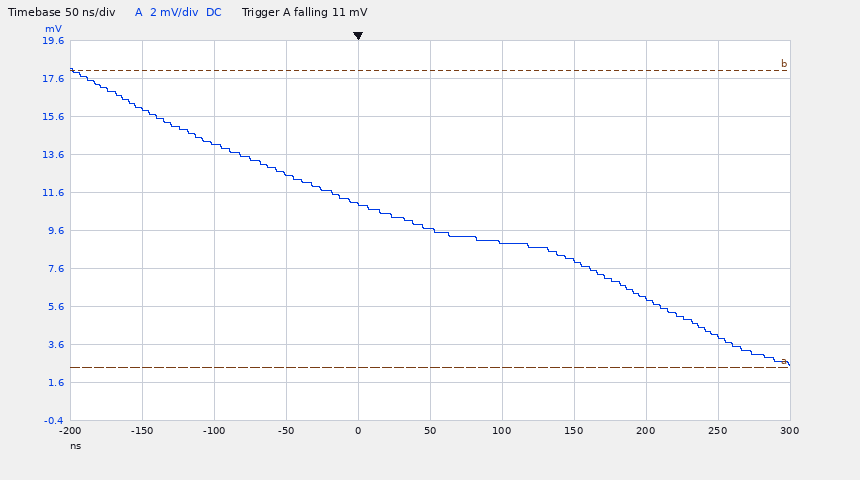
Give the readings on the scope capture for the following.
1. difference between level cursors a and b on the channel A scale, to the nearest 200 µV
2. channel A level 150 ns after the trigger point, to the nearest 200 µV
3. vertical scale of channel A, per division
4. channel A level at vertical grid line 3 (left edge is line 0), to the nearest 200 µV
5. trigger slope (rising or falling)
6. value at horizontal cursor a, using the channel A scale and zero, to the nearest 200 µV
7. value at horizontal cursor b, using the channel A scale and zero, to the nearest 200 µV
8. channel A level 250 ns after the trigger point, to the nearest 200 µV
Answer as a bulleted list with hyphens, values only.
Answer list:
- 15.6 mV
- 8.0 mV
- 2 mV
- 12.6 mV
- falling
- 2.4 mV
- 18.0 mV
- 4.0 mV
